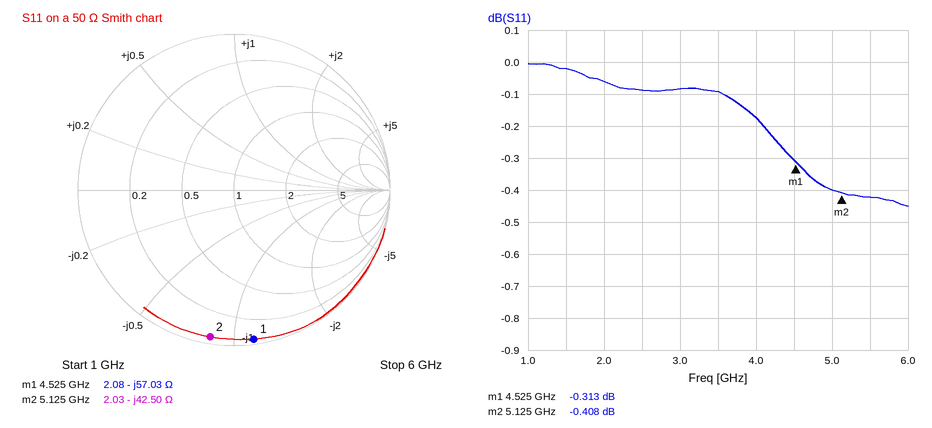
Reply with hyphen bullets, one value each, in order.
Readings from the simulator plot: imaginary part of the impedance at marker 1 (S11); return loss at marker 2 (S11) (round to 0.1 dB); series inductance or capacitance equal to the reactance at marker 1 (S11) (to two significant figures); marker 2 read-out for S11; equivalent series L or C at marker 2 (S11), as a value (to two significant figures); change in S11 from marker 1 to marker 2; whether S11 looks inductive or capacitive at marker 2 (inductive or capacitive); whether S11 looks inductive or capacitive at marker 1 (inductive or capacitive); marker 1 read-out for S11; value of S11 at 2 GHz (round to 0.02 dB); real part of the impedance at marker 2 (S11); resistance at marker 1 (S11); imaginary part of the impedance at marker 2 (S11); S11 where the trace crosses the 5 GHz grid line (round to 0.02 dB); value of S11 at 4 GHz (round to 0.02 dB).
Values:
- -57.03 Ω
- 0.4 dB
- 620 fF
- -0.408 dB
- 730 fF
- -0.095 dB
- capacitive
- capacitive
- -0.313 dB
- -0.06 dB
- 2.03 Ω
- 2.08 Ω
- -42.50 Ω
- -0.40 dB
- -0.18 dB
